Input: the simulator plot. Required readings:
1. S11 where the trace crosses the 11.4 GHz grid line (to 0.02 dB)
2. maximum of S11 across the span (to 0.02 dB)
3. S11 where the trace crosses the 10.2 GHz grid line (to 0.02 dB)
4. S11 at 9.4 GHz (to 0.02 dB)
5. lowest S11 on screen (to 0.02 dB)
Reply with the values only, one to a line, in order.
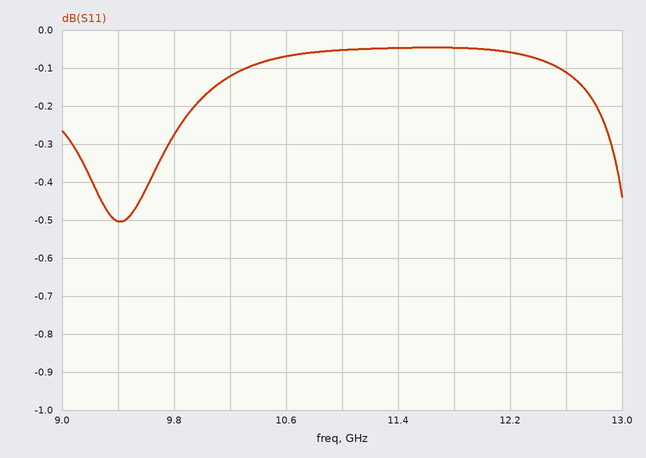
-0.04 dB
-0.04 dB
-0.12 dB
-0.50 dB
-0.50 dB
